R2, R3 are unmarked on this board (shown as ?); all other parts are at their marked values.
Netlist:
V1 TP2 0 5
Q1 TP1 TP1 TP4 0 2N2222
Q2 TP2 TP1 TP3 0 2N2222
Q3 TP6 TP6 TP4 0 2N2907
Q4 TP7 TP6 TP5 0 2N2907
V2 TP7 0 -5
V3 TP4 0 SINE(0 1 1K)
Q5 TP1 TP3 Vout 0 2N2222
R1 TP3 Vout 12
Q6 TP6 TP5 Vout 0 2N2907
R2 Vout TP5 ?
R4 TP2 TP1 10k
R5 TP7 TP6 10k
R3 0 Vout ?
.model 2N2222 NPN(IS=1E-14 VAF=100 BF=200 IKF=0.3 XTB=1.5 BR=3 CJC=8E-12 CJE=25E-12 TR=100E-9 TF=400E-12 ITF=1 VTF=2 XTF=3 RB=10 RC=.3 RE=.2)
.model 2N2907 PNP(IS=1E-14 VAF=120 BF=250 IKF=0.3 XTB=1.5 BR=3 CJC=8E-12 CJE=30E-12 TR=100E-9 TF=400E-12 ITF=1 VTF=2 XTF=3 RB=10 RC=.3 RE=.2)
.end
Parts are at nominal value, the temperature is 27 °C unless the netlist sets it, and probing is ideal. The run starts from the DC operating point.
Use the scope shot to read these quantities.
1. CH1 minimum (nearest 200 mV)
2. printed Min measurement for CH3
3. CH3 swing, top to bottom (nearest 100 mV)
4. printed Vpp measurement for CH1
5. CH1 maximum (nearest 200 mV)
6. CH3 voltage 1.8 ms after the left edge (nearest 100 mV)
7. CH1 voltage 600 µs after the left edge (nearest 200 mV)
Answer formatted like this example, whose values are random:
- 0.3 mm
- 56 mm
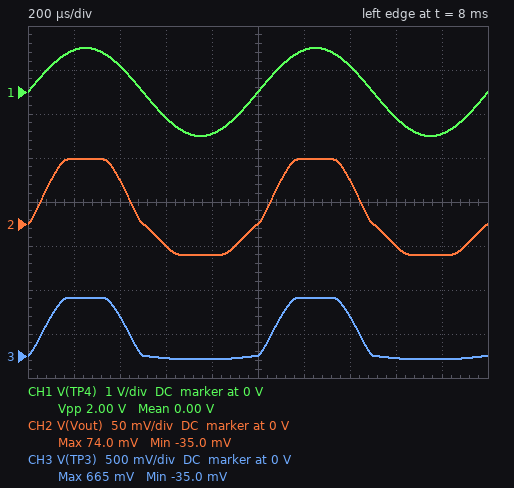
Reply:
- -1.0 V
- -35.0 mV
- 700 mV
- 2.00 V
- 1.0 V
- 0 V
- -600 mV
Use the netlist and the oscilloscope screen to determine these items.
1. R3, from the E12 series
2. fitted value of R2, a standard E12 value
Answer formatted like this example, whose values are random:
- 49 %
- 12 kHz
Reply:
- 1.5 Ω
- 27 Ω
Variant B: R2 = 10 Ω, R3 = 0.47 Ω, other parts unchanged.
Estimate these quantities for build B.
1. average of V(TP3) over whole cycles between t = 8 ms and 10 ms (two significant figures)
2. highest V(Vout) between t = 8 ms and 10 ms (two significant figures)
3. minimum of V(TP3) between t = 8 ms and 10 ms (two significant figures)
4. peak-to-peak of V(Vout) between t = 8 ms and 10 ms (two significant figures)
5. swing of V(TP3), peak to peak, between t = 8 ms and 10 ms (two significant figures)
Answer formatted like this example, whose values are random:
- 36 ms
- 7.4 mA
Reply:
- 210 mV
- 23 mV
- -28 mV
- 51 mV
- 640 mV
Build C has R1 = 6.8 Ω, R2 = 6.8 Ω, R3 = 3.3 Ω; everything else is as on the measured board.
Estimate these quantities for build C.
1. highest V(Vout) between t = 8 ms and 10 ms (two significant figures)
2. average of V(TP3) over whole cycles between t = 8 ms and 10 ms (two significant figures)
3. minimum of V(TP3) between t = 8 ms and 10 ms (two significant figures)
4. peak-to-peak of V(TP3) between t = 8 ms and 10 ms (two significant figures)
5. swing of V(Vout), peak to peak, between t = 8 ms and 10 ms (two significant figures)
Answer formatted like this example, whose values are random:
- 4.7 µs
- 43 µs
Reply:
- 210 mV
- 140 mV
- -240 mV
- 870 mV
- 440 mV
